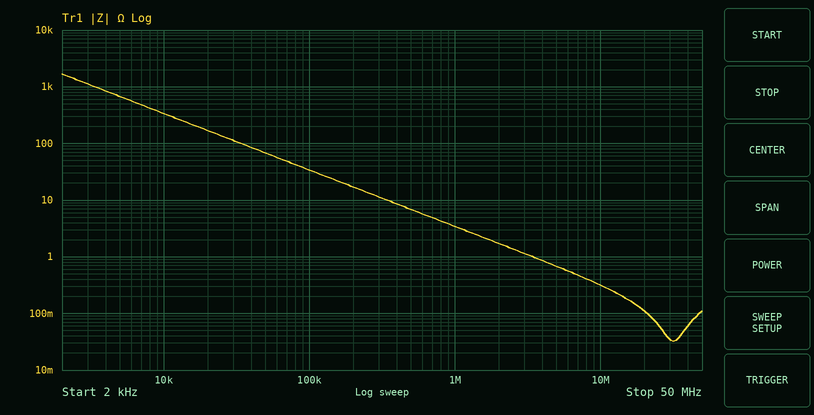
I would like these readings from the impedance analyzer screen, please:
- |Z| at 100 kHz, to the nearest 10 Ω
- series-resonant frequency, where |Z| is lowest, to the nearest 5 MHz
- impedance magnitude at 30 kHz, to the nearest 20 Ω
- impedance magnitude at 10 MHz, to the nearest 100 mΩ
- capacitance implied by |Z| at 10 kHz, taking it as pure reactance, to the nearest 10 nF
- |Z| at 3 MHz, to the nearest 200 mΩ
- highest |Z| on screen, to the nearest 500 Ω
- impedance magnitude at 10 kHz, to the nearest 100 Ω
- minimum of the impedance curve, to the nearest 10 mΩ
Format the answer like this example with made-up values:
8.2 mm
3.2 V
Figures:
30 Ω
30 MHz
120 Ω
300 mΩ
50 nF
1.2 Ω
1.5 kΩ
300 Ω
30 mΩ
